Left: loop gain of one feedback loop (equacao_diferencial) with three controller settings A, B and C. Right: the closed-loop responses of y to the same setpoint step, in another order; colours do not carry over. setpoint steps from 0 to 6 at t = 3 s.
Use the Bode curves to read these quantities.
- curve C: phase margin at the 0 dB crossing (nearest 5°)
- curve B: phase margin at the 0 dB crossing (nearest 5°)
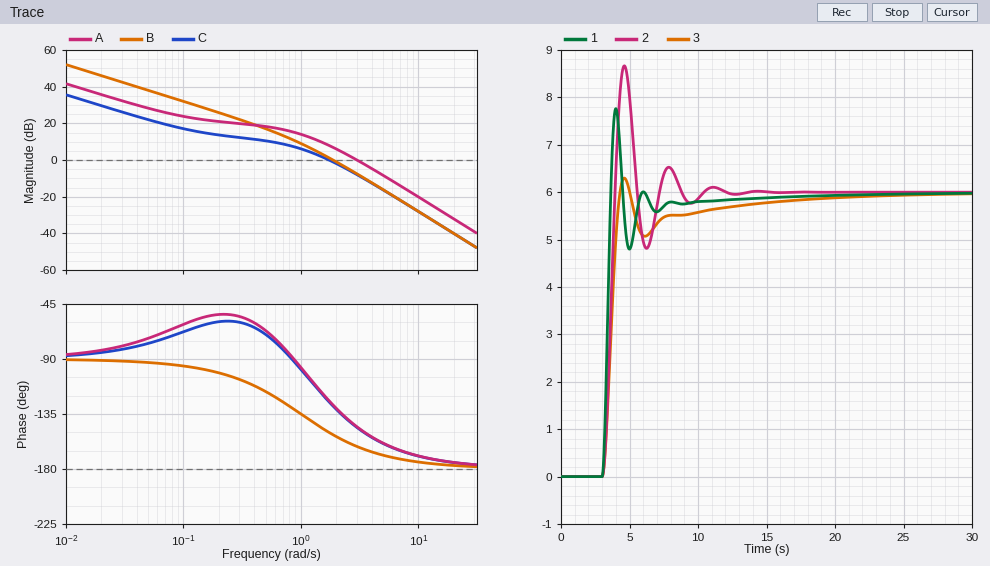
55°
30°
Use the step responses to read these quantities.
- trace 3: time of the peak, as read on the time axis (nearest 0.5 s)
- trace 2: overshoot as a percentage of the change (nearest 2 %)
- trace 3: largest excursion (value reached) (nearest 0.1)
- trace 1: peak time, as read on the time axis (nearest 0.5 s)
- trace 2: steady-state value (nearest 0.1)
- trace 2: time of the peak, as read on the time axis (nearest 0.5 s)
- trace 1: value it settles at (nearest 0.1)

4.5 s
44 %
6.3
4.0 s
6.0
4.5 s
6.0
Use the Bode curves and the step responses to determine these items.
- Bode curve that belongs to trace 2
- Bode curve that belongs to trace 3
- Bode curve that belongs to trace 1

B
C
A
